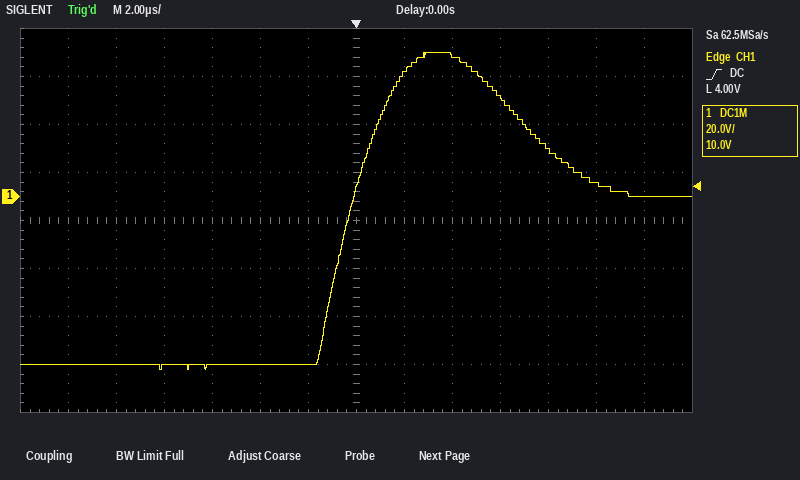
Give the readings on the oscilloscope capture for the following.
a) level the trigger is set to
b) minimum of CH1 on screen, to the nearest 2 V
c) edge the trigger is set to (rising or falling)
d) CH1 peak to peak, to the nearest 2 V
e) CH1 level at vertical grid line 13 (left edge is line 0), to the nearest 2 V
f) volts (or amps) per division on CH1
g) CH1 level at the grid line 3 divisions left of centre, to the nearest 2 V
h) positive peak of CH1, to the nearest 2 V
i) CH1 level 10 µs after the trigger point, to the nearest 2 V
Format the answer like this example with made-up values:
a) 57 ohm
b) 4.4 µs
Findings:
a) 4.00 V
b) -72 V
c) rising
d) 132 V
e) 0 V
f) 20 V
g) -70 V
h) 60 V
i) 6 V
